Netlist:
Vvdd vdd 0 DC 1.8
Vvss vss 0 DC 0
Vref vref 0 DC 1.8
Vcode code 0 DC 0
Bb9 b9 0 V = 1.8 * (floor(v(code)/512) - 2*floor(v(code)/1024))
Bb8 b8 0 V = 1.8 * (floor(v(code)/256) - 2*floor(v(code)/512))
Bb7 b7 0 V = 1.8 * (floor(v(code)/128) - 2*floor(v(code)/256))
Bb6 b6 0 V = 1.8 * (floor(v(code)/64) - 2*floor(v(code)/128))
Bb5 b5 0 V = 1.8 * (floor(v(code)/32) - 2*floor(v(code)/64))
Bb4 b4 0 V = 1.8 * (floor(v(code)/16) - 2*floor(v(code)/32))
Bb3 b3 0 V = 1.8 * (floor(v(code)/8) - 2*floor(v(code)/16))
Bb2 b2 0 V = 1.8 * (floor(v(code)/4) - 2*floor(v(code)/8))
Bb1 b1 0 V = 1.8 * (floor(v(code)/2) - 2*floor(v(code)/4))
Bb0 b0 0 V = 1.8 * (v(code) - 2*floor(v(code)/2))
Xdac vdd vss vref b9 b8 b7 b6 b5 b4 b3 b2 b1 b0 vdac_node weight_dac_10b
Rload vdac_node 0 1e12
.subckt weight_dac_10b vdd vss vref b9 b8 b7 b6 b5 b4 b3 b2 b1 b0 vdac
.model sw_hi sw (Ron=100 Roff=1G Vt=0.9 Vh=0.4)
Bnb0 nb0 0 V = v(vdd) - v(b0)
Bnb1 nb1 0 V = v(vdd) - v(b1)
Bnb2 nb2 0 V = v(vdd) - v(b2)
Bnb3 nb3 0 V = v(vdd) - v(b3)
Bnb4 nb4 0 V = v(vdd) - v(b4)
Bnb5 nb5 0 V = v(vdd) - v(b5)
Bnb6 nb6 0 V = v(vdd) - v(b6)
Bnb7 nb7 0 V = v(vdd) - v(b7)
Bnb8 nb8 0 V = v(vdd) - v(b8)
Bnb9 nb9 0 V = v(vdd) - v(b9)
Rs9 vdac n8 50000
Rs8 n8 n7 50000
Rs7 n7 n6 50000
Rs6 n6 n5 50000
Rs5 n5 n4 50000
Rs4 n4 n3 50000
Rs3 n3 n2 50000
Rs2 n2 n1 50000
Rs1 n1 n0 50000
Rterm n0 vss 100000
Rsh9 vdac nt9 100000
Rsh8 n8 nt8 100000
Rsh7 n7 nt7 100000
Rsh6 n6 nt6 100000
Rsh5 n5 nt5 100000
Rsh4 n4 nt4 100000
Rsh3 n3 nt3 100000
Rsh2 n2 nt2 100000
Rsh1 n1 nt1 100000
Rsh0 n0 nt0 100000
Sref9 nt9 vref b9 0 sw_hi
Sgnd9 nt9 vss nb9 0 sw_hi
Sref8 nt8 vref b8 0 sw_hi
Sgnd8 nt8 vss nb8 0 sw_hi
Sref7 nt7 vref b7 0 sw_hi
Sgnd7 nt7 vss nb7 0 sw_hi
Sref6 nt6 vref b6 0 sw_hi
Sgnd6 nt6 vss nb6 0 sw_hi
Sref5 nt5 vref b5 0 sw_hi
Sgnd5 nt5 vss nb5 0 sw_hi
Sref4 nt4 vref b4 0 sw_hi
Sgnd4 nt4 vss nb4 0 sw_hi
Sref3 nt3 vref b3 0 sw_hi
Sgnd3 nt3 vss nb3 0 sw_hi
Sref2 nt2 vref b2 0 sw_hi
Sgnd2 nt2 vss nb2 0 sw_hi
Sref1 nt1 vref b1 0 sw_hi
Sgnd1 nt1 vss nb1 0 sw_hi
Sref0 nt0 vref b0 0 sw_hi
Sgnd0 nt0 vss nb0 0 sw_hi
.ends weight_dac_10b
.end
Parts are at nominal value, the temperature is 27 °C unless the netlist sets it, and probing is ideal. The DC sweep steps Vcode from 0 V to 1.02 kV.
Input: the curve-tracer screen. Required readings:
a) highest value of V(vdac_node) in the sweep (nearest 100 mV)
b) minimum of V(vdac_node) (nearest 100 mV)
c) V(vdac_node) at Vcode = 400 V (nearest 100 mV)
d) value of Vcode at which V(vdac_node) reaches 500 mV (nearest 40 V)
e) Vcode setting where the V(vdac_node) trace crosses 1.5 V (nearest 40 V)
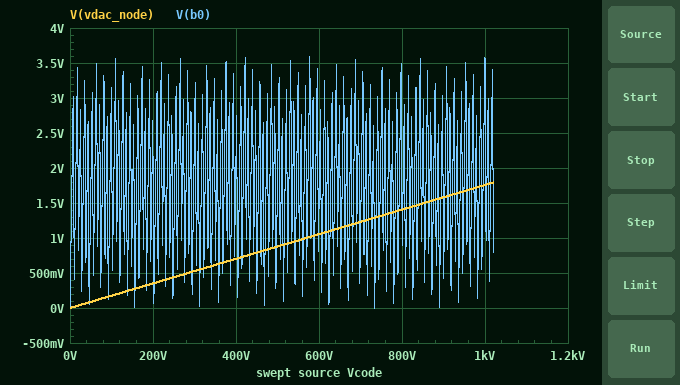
1.8 V
0 V
700 mV
280 V
840 V
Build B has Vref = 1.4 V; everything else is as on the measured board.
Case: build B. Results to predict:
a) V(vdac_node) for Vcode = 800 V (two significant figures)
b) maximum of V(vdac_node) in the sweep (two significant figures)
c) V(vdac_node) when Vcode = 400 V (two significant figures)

1.1 V
1.4 V
550 mV
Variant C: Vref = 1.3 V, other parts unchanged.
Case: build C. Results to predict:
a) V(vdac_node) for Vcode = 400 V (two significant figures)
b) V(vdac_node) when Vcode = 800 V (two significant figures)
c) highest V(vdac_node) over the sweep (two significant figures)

510 mV
1.0 V
1.3 V
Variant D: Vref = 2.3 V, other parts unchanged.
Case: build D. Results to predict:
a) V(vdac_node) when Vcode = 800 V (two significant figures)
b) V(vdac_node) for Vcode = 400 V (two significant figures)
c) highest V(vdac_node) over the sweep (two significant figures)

1.8 V
900 mV
2.3 V
